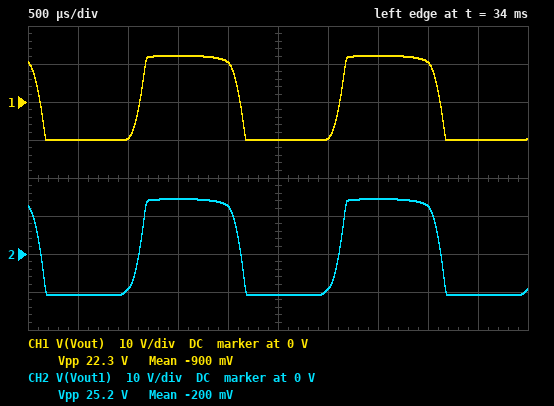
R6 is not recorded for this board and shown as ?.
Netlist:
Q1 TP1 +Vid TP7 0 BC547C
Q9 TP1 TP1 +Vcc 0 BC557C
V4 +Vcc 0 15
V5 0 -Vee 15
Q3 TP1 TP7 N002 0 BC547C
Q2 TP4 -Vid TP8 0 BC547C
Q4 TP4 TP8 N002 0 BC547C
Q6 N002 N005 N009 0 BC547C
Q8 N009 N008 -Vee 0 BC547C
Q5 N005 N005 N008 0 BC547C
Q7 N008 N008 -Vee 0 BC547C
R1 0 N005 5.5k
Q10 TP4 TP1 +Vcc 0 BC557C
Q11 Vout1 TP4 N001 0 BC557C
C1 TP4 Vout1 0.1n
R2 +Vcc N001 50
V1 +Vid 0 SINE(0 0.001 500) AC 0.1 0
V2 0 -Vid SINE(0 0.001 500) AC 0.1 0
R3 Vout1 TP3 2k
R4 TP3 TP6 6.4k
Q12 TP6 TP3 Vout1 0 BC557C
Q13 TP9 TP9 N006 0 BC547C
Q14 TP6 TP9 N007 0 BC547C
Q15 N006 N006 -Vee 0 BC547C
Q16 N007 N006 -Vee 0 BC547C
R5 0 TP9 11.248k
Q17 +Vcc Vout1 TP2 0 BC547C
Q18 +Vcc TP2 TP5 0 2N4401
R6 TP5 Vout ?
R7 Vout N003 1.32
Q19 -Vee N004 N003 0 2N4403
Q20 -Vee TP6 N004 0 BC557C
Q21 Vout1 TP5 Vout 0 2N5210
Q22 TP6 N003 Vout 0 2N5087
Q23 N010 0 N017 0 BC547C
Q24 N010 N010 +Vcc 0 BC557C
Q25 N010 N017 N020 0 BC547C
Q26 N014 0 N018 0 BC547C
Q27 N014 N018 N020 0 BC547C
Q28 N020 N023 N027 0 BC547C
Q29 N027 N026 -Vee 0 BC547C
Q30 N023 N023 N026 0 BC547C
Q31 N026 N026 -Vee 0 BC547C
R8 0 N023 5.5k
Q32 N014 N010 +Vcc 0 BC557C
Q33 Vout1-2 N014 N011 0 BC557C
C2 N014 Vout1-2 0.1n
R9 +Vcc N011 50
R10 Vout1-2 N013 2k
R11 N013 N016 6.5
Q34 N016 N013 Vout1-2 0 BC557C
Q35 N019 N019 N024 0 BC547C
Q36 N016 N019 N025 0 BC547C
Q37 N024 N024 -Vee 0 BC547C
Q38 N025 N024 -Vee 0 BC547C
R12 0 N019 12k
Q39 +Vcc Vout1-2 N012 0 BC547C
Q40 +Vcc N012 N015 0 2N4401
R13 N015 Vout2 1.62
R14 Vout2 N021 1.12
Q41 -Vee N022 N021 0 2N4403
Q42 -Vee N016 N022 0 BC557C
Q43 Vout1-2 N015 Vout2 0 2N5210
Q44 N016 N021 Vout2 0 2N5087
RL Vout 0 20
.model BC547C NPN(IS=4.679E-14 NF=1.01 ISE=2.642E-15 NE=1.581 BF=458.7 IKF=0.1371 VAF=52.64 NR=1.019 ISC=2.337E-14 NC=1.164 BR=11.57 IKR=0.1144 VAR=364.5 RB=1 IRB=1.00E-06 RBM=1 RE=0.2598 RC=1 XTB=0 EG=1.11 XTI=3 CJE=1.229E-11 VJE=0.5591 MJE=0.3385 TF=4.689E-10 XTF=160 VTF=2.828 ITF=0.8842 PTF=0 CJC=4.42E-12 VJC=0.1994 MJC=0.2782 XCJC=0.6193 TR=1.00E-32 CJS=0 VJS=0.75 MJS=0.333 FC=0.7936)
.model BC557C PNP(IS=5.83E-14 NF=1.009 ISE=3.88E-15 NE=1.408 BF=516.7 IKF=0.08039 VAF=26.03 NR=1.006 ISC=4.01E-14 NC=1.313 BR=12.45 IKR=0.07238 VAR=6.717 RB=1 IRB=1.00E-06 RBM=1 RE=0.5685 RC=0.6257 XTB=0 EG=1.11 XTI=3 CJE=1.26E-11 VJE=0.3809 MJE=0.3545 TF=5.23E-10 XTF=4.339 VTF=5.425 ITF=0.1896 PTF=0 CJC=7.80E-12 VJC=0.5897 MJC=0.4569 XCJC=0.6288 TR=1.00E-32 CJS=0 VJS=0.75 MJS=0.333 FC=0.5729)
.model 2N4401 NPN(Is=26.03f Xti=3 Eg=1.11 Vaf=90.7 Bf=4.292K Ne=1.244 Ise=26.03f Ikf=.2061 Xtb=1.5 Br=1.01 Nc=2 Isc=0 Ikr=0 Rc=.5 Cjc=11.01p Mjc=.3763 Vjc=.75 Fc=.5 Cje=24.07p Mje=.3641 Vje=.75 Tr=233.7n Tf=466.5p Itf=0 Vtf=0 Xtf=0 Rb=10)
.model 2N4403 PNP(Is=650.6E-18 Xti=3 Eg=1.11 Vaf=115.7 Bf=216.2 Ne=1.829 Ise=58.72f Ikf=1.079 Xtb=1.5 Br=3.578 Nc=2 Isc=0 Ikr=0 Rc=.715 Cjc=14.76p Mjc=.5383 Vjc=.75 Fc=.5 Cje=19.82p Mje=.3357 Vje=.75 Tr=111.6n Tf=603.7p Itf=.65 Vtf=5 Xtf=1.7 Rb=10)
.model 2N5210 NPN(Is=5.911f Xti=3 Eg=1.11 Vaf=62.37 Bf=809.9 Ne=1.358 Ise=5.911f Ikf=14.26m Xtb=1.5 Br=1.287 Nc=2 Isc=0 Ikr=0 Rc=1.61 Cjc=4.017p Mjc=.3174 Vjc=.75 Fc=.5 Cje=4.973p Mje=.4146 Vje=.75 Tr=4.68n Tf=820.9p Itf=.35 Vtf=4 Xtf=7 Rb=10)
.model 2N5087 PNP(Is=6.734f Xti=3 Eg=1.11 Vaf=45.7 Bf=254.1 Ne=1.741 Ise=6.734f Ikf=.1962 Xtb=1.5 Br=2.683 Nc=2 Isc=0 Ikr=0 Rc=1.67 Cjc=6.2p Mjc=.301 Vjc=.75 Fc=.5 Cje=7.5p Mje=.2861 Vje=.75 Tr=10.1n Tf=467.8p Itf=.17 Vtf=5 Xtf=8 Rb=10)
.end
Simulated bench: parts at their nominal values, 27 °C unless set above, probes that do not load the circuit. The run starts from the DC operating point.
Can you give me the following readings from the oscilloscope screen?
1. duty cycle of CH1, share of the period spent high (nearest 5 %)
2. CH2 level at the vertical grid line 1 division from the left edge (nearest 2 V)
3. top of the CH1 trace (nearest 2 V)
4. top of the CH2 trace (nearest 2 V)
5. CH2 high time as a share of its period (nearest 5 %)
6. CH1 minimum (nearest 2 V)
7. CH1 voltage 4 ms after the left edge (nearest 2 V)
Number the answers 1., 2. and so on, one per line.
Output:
1. 50 %
2. -10 V
3. 12 V
4. 14 V
5. 50 %
6. -10 V
7. 10 V
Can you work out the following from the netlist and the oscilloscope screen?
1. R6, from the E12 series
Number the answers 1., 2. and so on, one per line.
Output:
1. 1.2 Ω
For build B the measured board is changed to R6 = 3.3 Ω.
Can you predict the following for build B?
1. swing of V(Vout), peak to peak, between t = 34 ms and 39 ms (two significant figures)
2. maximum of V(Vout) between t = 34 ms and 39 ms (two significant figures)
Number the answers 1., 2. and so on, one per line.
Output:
1. 15 V
2. 4.6 V
